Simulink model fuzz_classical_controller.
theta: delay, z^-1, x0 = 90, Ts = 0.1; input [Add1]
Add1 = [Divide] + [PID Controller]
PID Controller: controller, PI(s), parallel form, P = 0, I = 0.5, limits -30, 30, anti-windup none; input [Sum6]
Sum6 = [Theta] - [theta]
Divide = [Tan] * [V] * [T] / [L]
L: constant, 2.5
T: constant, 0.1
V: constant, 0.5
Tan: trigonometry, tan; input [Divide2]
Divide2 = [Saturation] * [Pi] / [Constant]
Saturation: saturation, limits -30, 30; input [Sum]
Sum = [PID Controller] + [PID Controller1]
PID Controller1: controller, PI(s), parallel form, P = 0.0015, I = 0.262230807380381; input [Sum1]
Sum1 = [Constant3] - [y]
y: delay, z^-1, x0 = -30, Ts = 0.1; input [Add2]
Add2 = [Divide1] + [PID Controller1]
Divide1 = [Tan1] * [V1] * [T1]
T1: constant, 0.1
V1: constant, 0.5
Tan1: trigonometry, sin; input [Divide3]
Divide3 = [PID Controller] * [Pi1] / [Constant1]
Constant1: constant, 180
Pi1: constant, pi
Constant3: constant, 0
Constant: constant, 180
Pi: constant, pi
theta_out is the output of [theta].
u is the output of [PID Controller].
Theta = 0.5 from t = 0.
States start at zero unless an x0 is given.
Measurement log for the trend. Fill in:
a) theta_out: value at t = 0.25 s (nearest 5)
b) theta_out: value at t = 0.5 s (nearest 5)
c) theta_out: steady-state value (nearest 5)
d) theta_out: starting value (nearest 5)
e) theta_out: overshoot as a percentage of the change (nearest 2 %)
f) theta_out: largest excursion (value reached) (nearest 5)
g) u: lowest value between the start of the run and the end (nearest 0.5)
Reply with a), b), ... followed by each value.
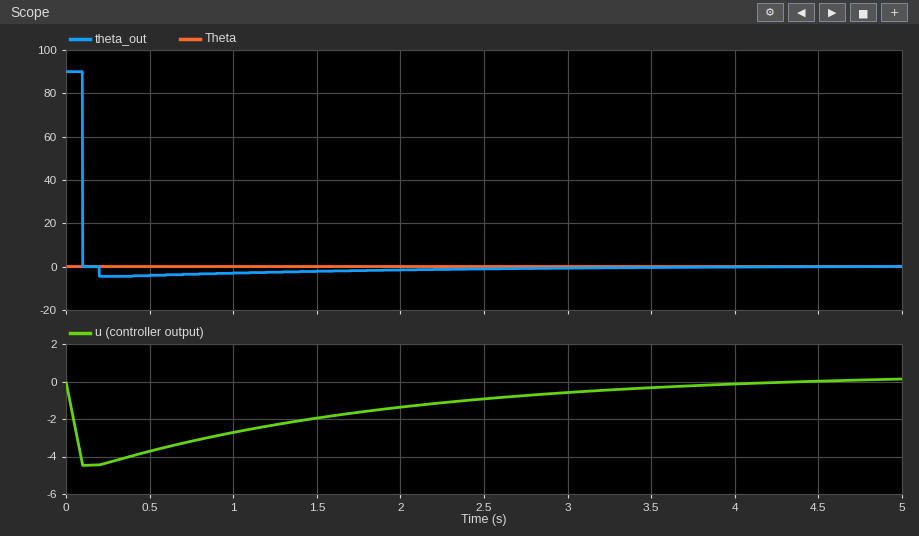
a) -5
b) -5
c) 0
d) 90
e) 6 %
f) -5
g) -4.5
